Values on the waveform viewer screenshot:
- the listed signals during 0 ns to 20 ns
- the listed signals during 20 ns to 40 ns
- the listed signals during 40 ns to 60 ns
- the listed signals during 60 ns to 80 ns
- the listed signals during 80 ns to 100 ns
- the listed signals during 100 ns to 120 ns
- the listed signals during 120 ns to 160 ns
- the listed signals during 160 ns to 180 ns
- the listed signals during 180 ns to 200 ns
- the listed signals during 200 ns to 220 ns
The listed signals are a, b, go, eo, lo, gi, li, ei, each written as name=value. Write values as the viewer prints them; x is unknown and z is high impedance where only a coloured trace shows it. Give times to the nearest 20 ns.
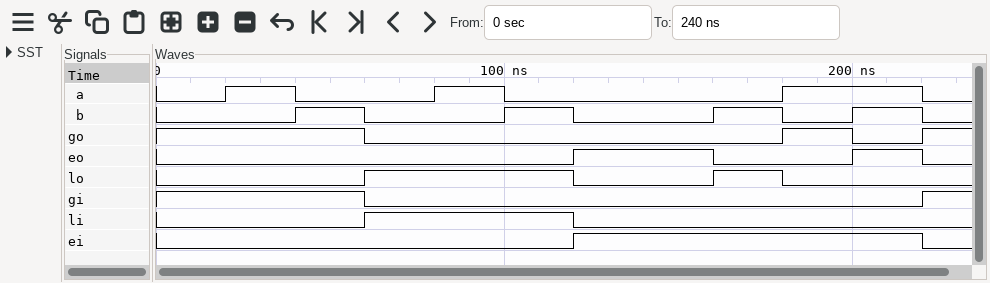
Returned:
a=0, b=0, go=1, eo=0, lo=0, gi=1, li=0, ei=0
a=1, b=0, go=1, eo=0, lo=0, gi=1, li=0, ei=0
a=0, b=1, go=1, eo=0, lo=0, gi=1, li=0, ei=0
a=0, b=0, go=0, eo=0, lo=1, gi=0, li=1, ei=0
a=1, b=0, go=0, eo=0, lo=1, gi=0, li=1, ei=0
a=0, b=1, go=0, eo=0, lo=1, gi=0, li=1, ei=0
a=0, b=0, go=0, eo=1, lo=0, gi=0, li=0, ei=1
a=0, b=1, go=0, eo=0, lo=1, gi=0, li=0, ei=1
a=1, b=0, go=1, eo=0, lo=0, gi=0, li=0, ei=1
a=1, b=1, go=0, eo=1, lo=0, gi=0, li=0, ei=1
